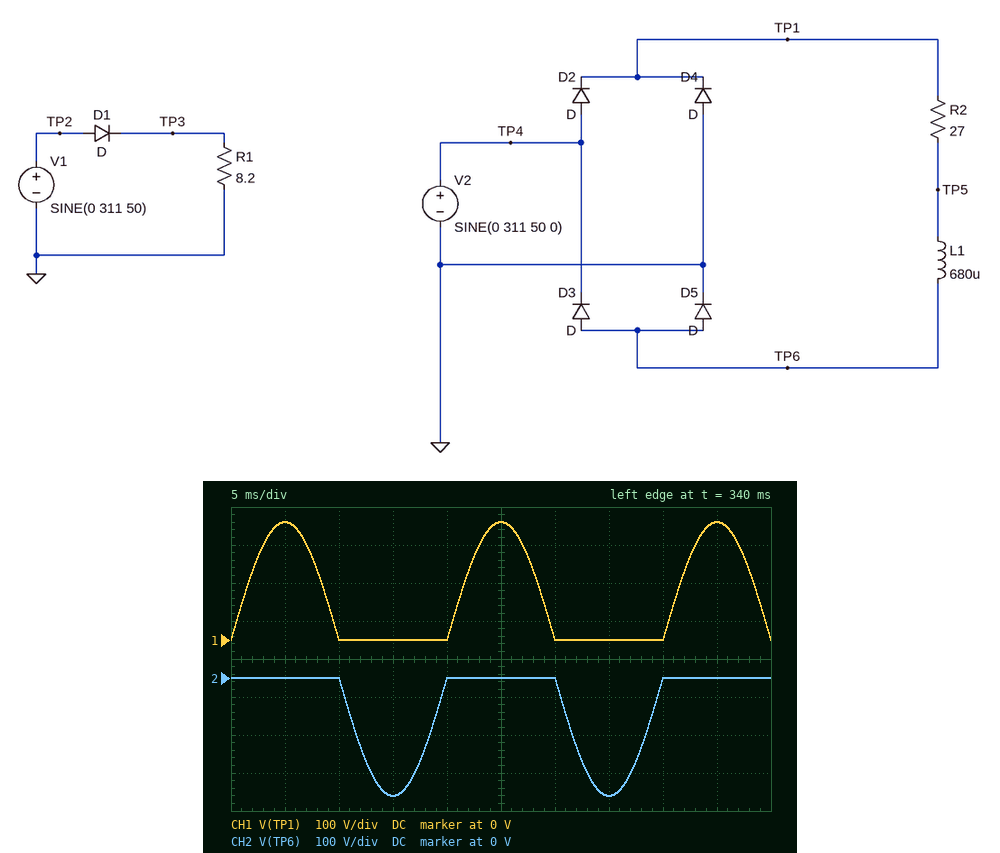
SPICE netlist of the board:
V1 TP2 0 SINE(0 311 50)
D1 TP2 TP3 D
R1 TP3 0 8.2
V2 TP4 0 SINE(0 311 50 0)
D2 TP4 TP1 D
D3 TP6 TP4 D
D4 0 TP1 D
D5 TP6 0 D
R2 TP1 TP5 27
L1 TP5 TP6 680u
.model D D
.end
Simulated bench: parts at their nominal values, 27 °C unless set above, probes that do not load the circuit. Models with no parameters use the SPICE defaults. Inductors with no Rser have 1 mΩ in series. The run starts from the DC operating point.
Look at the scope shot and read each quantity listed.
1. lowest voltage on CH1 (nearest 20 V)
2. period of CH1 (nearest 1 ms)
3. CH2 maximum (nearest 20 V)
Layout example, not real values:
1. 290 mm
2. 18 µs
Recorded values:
1. 0 V
2. 20 ms
3. 0 V
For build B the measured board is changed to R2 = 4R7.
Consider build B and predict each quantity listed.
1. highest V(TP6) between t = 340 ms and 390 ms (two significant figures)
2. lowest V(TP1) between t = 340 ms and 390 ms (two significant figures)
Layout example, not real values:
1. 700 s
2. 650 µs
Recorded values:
1. 940 mV
2. -940 mV
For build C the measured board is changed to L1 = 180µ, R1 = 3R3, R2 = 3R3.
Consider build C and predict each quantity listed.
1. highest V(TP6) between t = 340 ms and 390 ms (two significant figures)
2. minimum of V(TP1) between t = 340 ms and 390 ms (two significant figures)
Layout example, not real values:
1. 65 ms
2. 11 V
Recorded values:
1. 950 mV
2. -950 mV
